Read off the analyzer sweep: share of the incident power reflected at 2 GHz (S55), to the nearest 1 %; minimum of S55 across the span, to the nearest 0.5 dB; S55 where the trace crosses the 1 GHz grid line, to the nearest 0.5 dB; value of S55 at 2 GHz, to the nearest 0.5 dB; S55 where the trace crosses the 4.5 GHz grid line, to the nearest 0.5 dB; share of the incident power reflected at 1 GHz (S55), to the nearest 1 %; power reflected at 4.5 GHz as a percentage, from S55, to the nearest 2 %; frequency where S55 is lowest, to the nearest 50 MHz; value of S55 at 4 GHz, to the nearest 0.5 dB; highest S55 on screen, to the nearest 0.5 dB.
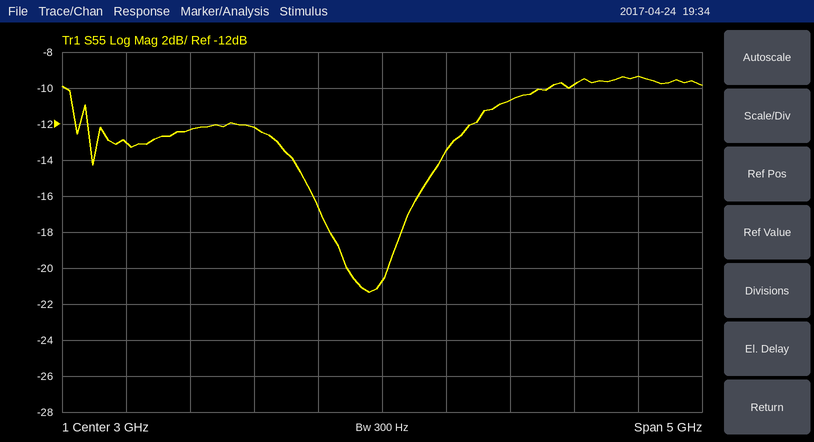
6 %
-21.5 dB
-13.0 dB
-12.0 dB
-10.0 dB
5 %
10 %
2.90 GHz
-10.5 dB
-9.5 dB
